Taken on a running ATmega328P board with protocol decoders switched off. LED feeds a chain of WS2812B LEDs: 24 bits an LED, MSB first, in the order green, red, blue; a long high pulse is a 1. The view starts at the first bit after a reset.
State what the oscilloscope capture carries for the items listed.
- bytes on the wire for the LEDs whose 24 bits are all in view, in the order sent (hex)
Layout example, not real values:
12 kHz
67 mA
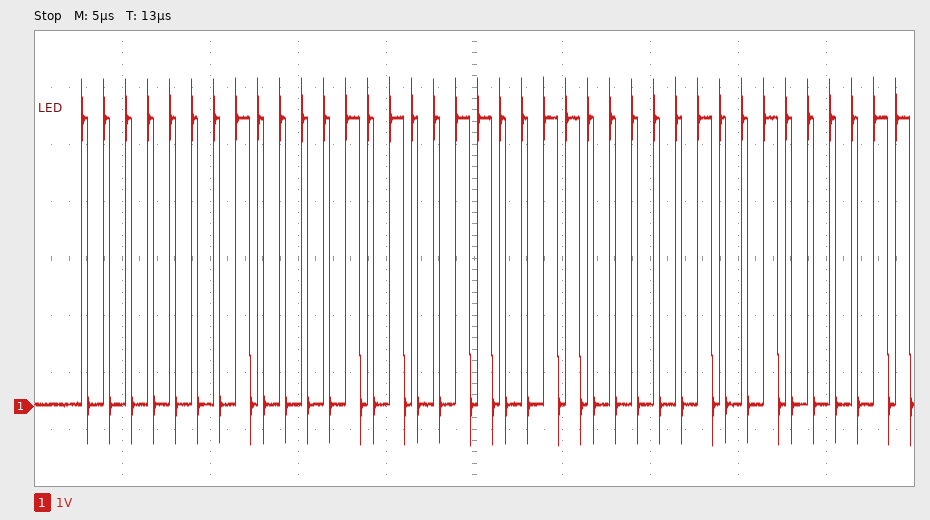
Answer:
01 0A 66
